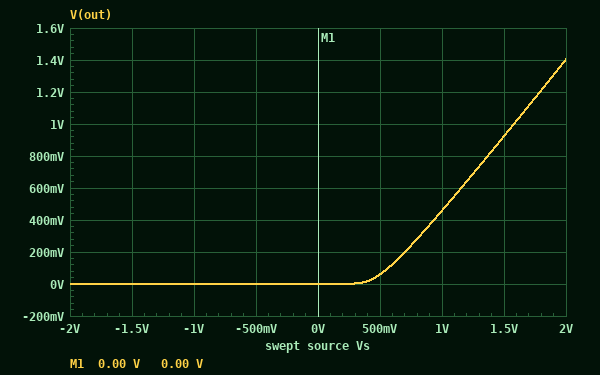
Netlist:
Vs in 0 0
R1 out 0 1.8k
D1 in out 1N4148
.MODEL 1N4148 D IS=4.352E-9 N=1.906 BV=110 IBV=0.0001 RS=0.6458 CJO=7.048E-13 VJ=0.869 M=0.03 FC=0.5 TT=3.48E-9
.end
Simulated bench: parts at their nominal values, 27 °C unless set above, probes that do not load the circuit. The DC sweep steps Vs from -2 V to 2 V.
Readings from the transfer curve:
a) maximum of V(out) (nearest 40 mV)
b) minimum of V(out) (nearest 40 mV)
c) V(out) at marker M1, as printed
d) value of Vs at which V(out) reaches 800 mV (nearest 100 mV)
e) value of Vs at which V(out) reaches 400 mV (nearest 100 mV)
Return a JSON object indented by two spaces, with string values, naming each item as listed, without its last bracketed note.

{
  "maximum of V(out)": "1.40 V",
  "minimum of V(out)": "0 V",
  "V(out) at marker M1, as printed": "0.00 V",
  "value of Vs at which V(out) reaches 800 mV": "1.4 V",
  "value of Vs at which V(out) reaches 400 mV": "900 mV"
}
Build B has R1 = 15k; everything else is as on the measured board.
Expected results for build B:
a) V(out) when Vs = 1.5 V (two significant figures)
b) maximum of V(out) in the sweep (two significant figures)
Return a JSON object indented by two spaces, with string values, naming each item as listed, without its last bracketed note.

{
  "V(out) when Vs = 1.5 V": "1.0 V",
  "maximum of V(out) in the sweep": "1.5 V"
}
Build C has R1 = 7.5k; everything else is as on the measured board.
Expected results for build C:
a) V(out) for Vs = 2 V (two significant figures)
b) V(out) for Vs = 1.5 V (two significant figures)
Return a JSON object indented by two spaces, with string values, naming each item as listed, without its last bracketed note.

{
  "V(out) for Vs = 2 V": "1.5 V",
  "V(out) for Vs = 1.5 V": "990 mV"
}
